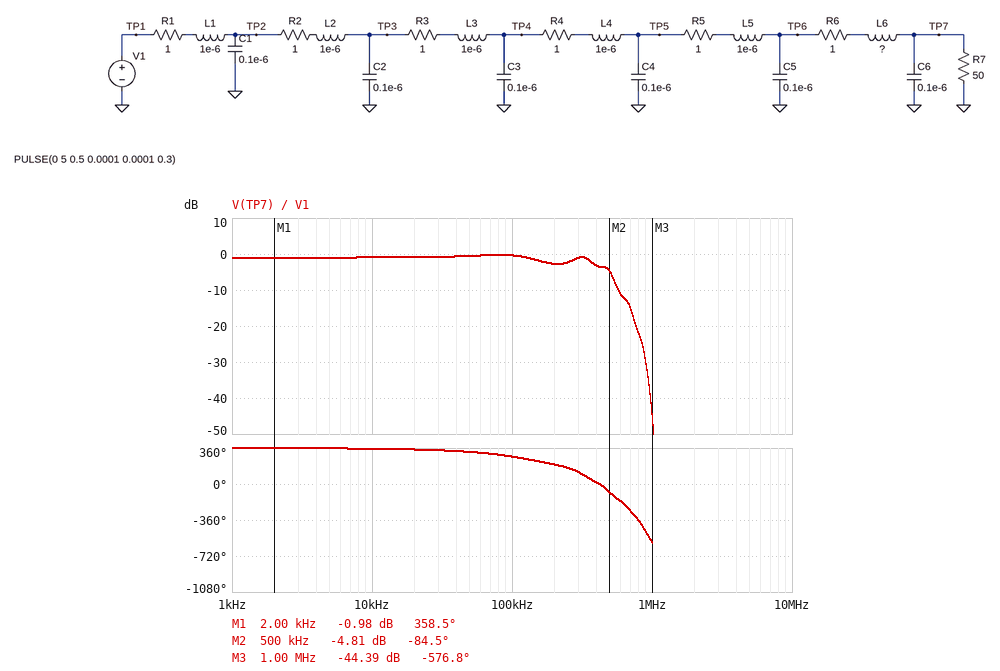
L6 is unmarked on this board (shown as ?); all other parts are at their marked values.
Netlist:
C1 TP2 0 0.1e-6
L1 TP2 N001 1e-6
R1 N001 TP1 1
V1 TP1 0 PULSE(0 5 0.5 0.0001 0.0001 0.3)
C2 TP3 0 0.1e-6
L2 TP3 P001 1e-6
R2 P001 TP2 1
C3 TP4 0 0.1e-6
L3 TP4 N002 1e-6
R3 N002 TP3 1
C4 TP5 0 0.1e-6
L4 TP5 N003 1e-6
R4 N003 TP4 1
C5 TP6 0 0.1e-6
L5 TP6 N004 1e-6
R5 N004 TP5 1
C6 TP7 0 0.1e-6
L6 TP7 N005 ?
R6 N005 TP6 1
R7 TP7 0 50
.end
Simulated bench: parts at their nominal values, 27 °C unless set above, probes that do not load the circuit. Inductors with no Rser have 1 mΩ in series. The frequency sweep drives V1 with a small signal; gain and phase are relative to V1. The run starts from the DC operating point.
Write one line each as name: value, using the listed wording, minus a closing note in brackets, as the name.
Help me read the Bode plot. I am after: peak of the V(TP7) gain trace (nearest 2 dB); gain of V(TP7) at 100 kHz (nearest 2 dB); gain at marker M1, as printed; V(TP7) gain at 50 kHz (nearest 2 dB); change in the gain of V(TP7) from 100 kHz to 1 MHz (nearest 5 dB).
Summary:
peak of the V(TP7) gain trace: 0 dB
gain of V(TP7) at 100 kHz: 0 dB
gain at marker M1, as printed: -0.98 dB
V(TP7) gain at 50 kHz: 0 dB
change in the gain of V(TP7) from 100 kHz to 1 MHz: -45 dB
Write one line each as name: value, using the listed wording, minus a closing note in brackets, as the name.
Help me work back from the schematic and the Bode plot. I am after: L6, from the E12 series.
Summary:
L6, from the E12 series: 2.2 µH
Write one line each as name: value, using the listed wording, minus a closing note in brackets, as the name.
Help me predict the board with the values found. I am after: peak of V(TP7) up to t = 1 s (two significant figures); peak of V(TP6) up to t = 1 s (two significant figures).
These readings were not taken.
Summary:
peak of V(TP7) up to t = 1 s: 4.5 V
peak of V(TP6) up to t = 1 s: 4.6 V
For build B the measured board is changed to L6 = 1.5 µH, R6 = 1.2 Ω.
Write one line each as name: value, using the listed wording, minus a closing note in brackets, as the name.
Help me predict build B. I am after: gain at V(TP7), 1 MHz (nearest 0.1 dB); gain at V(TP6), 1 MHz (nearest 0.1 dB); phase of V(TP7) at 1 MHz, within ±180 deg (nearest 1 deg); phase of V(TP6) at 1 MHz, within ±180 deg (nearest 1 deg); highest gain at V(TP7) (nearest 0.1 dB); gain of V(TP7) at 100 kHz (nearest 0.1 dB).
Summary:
gain at V(TP7), 1 MHz: -39.6 dB
gain at V(TP6), 1 MHz: -25.6 dB
phase of V(TP7) at 1 MHz, within ±180 deg: 152 deg
phase of V(TP6) at 1 MHz, within ±180 deg: -39 deg
highest gain at V(TP7): -0.4 dB
gain of V(TP7) at 100 kHz: -0.6 dB
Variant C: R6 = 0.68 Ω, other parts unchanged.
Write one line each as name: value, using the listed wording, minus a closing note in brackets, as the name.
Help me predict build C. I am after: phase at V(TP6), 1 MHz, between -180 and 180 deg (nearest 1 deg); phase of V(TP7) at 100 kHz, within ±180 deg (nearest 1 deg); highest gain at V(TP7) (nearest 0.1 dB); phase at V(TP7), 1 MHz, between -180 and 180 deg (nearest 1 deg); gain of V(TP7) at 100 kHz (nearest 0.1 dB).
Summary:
phase at V(TP6), 1 MHz, between -180 and 180 deg: -44 deg
phase of V(TP7) at 100 kHz, within ±180 deg: -85 deg
highest gain at V(TP7): -0.2 dB
phase at V(TP7), 1 MHz, between -180 and 180 deg: 141 deg
gain of V(TP7) at 100 kHz: -0.3 dB
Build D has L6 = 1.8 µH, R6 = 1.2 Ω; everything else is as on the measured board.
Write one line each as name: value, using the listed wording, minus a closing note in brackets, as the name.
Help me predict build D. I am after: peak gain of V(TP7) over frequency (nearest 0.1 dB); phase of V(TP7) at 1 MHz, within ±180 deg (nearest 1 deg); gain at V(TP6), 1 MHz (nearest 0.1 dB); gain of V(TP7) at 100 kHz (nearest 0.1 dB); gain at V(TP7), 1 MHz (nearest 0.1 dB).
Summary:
peak gain of V(TP7) over frequency: -0.4 dB
phase of V(TP7) at 1 MHz, within ±180 deg: 148 deg
gain at V(TP6), 1 MHz: -26.2 dB
gain of V(TP7) at 100 kHz: -0.5 dB
gain at V(TP7), 1 MHz: -42.0 dB
